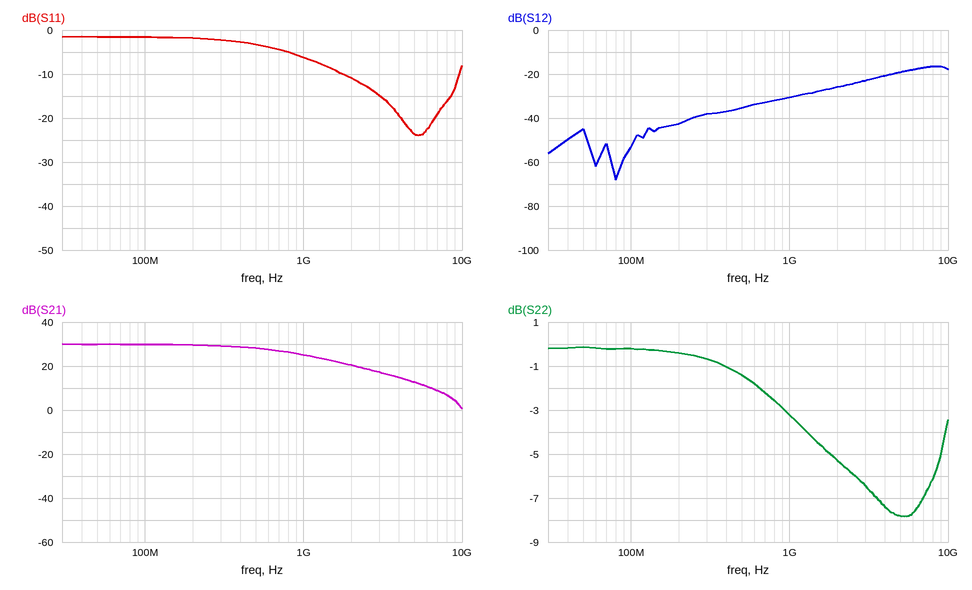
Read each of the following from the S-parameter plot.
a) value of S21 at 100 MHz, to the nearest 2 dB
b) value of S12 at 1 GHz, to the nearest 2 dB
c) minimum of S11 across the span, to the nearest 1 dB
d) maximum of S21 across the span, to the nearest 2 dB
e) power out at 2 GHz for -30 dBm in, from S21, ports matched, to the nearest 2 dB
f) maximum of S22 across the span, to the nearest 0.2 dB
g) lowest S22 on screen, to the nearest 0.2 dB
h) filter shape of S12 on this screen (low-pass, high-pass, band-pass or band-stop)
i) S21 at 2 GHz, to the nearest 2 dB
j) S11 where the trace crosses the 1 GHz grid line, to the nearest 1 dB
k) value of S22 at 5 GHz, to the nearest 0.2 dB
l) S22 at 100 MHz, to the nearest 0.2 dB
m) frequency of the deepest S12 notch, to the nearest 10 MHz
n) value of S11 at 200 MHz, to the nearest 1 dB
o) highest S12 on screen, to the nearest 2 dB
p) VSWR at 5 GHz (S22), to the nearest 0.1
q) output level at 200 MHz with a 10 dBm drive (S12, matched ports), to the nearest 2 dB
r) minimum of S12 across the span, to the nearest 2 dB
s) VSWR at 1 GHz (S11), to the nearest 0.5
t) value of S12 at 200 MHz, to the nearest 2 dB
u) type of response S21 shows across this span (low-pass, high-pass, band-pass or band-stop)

30 dB
-30 dB
-24 dB
30 dB
-10 dBm
-0.2 dB
-7.8 dB
high-pass
20 dB
-6 dB
-7.8 dB
-0.2 dB
80 MHz
-2 dB
-16 dB
2.4
-32 dBm
-68 dB
3.0
-42 dB
low-pass
